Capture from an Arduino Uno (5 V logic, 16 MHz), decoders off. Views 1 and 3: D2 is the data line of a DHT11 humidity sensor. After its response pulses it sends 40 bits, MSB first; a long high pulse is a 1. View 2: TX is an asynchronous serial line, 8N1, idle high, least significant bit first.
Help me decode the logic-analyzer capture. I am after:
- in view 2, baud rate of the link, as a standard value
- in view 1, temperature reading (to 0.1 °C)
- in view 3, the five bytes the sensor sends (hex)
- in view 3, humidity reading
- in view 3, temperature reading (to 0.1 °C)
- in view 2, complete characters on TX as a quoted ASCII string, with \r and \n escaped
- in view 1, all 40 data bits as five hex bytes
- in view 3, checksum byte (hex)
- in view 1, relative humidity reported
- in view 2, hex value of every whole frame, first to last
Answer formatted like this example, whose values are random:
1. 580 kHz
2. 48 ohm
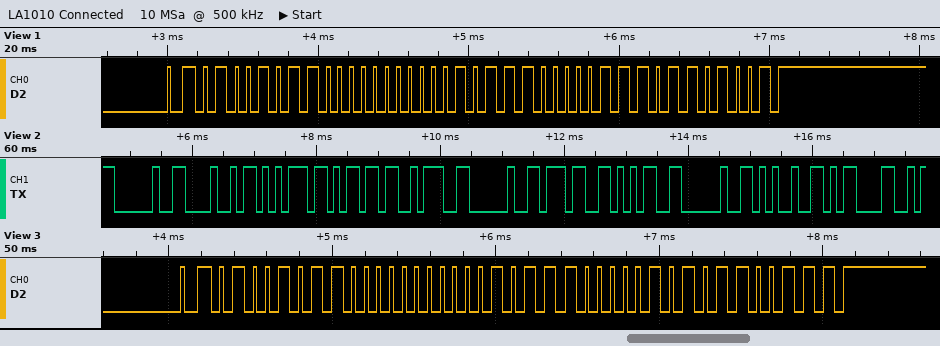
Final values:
1. 9600 baud
2. 23.7 °C
3. 4B 00 17 05 67
4. 75 %
5. 23.5 °C
6. " Hum: 75 %\r"
7. 4B 00 17 07 69
8. 0x67
9. 75 %
10. 20 48 75 6D 3A 20 37 35 20 25 0D
